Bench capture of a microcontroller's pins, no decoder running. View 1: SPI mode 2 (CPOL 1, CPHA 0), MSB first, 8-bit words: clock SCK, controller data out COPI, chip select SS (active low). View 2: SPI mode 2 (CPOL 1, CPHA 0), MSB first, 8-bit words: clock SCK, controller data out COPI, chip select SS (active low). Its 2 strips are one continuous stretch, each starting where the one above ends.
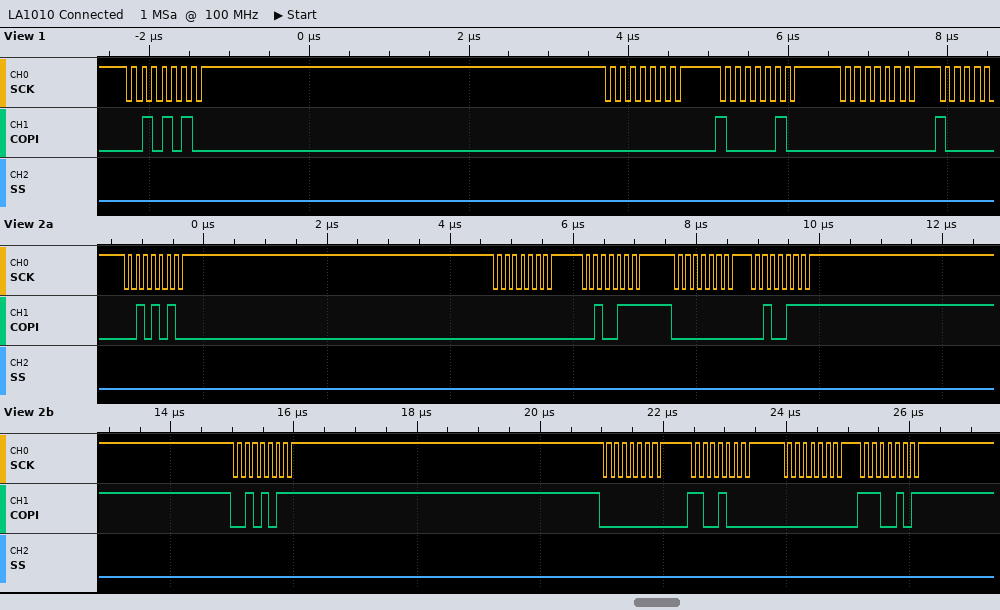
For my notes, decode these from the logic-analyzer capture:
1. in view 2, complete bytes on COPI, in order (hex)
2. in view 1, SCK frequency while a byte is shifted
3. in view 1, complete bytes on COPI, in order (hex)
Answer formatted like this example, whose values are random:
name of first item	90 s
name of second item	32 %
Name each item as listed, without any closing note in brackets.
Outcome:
in view 2, complete bytes on COPI, in order	2A 00 27 00 27 2B 00 C8 00 E5
in view 1, SCK frequency while a byte is shifted	8 MHz
in view 1, complete bytes on COPI, in order	2A 00 82 00
